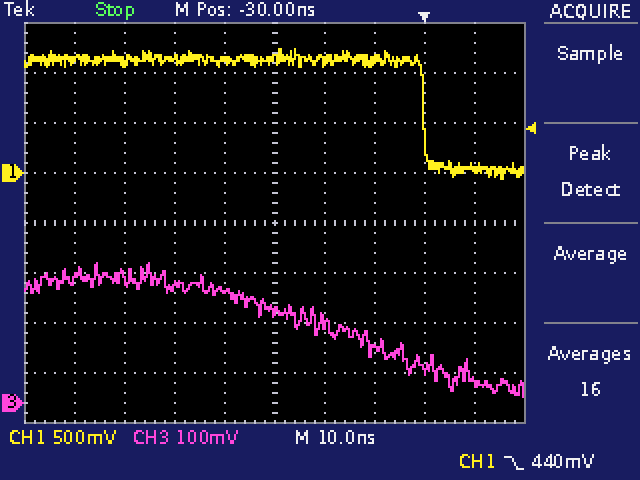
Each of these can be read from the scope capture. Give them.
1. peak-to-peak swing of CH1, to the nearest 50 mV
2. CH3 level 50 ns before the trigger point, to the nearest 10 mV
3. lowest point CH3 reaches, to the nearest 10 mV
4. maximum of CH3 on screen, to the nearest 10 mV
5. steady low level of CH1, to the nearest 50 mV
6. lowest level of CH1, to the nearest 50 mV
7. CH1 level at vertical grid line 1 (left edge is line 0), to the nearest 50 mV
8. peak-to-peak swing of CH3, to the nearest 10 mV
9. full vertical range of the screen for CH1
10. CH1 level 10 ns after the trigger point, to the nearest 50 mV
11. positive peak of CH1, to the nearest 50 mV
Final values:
1.30 V
230 mV
10 mV
280 mV
50 mV
-50 mV
1.15 V
270 mV
4 V
50 mV
1.25 V
